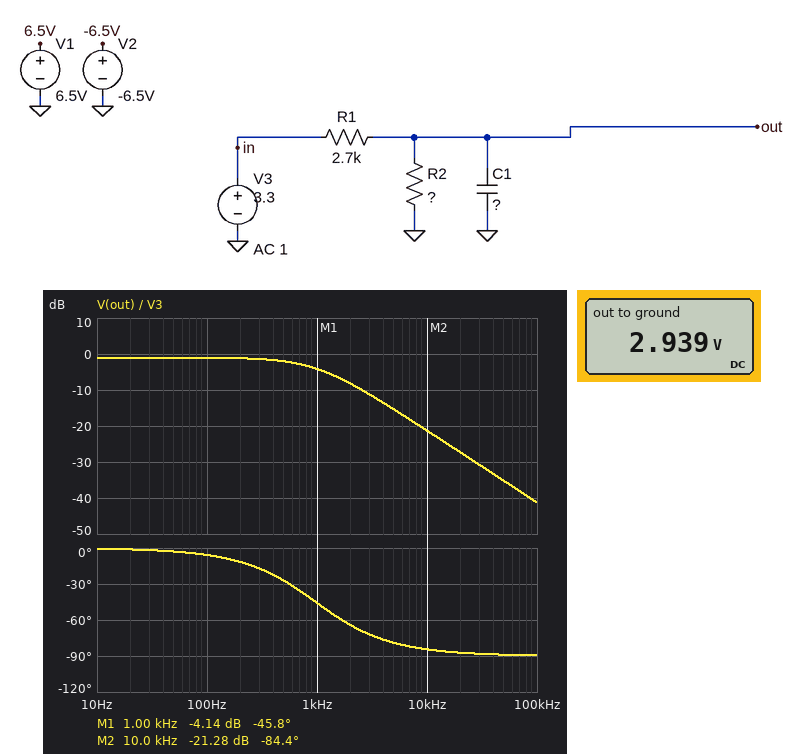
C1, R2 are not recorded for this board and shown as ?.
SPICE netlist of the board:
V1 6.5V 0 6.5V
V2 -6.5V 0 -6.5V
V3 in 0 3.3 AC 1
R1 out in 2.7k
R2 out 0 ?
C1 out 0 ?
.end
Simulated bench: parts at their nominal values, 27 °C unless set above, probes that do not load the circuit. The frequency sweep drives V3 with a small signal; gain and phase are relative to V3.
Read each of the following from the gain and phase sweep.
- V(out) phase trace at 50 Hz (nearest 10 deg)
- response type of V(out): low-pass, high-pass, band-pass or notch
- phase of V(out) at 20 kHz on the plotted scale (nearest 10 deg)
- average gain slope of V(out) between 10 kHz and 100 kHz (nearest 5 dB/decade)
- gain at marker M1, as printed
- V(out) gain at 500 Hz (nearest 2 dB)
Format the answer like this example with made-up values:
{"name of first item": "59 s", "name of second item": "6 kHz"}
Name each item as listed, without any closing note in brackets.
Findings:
{"V(out) phase trace at 50 Hz": "0 deg", "response type of V(out): low-pass, high-pass, band-pass or notch": "low-pass", "phase of V(out) at 20 kHz on the plotted scale": "-90 deg", "average gain slope of V(out) between 10 kHz and 100 kHz": "-20 dB/decade", "gain at marker M1, as printed": "-4.14 dB", "V(out) gain at 500 Hz": "-2 dB"}
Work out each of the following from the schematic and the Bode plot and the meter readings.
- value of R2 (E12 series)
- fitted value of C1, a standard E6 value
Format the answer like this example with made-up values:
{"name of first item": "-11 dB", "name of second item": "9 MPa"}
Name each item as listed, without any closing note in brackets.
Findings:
{"value of R2": "22 kΩ", "fitted value of C1, a standard E6 value": "68 nF"}
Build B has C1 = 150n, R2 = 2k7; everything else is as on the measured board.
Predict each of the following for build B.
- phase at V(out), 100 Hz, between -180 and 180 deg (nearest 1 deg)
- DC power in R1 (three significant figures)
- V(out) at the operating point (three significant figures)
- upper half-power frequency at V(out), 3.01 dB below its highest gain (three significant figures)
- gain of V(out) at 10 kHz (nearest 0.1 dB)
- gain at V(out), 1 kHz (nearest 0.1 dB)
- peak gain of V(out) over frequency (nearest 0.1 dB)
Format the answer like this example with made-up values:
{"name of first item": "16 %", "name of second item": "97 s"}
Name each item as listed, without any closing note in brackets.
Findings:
{"phase at V(out), 100 Hz, between -180 and 180 deg": "-7 deg", "DC power in R1": "1.01 mW", "V(out) at the operating point": "1.65 V", "upper half-power frequency at V(out), 3.01 dB below its highest gain": "786 Hz", "gain of V(out) at 10 kHz": "-28.1 dB", "gain at V(out), 1 kHz": "-10.2 dB", "peak gain of V(out) over frequency": "-6.0 dB"}
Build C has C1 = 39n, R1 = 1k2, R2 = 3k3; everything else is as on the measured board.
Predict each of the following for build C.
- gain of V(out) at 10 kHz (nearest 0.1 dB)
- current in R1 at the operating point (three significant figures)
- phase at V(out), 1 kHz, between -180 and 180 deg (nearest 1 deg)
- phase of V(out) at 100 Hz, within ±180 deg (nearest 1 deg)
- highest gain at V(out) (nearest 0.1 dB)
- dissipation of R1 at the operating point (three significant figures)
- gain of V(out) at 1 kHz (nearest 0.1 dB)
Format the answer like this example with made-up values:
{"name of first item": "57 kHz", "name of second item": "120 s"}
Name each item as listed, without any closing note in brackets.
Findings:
{"gain of V(out) at 10 kHz": "-10.2 dB", "current in R1 at the operating point": "733 µA", "phase at V(out), 1 kHz, between -180 and 180 deg": "-12 deg", "phase of V(out) at 100 Hz, within ±180 deg": "-1 deg", "highest gain at V(out)": "-2.7 dB", "dissipation of R1 at the operating point": "645 µW", "gain of V(out) at 1 kHz": "-2.9 dB"}
